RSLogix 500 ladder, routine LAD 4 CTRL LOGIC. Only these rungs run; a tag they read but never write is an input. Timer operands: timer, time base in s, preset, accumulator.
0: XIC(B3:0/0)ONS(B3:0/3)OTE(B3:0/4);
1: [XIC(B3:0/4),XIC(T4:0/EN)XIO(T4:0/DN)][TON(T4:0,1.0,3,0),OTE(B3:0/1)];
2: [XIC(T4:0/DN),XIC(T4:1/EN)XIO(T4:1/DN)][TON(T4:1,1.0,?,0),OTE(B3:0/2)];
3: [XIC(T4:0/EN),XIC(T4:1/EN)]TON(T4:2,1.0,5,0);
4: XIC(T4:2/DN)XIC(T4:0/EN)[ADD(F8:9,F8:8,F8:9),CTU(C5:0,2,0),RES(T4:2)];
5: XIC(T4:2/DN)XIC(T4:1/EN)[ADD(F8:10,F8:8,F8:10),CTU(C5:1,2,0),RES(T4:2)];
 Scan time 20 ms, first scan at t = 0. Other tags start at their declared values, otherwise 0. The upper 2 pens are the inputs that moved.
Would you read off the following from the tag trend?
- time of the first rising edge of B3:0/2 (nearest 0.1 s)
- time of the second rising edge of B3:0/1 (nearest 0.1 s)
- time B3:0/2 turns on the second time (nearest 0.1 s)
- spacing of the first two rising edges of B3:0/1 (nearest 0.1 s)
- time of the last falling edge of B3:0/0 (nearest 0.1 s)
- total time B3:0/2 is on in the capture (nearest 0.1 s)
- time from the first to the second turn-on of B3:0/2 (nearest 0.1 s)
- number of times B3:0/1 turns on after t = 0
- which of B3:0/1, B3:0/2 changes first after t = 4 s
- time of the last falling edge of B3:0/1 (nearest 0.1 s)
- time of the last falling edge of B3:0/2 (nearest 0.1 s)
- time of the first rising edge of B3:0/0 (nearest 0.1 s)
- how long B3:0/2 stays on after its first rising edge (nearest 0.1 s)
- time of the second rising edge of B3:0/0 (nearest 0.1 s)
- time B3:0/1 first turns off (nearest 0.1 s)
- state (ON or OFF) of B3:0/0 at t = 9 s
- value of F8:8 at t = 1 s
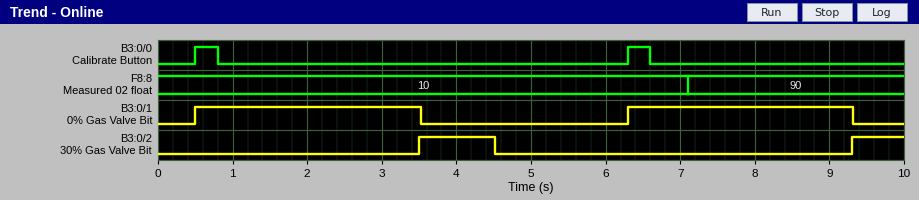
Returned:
3.5 s
6.3 s
9.3 s
5.8 s
6.6 s
1.7 s
5.8 s
2
B3:0/2
9.3 s
4.5 s
0.5 s
1.0 s
6.3 s
3.5 s
OFF
10
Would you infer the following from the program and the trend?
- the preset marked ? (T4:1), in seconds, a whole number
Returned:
1 s
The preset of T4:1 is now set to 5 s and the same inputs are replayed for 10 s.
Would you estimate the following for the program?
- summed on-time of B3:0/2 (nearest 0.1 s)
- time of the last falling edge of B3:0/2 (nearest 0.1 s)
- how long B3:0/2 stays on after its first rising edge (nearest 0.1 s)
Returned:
5.7 s
8.5 s
5.0 s
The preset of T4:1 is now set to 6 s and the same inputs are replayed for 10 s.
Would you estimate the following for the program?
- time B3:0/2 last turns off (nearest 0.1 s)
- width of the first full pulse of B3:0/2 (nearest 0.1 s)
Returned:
9.5 s
6.0 s
